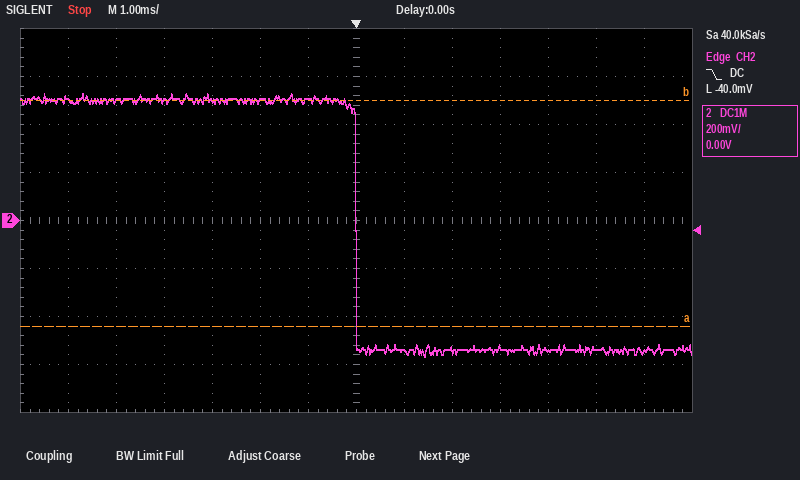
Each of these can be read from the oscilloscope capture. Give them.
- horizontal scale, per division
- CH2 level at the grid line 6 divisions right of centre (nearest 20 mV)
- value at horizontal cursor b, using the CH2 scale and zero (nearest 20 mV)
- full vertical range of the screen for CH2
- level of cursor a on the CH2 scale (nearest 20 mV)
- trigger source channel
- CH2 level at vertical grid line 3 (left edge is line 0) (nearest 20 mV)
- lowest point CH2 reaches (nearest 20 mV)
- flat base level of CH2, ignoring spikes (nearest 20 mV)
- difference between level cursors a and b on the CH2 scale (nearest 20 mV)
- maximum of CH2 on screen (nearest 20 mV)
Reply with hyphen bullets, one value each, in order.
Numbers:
- 1 ms
- -540 mV
- 500 mV
- 1.6 V
- -440 mV
- CH2
- 500 mV
- -560 mV
- -540 mV
- 940 mV
- 520 mV
